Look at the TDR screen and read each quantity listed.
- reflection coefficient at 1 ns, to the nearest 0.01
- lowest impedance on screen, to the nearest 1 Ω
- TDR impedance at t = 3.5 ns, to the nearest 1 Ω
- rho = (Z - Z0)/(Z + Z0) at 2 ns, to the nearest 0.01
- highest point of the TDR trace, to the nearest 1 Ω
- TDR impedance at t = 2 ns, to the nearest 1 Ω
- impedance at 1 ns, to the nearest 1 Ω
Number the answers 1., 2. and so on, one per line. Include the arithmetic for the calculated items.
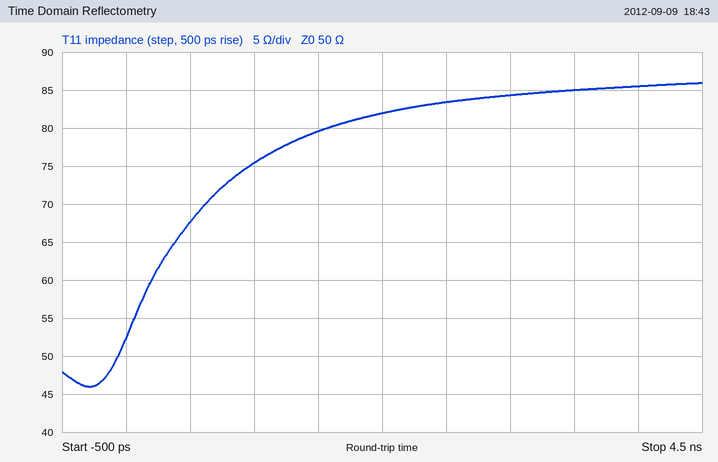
1. (75 − 50)/(75 + 50) ≈ +0.20
2. 46 Ω
3. 85 Ω
4. (82 − 50)/(82 + 50) ≈ +0.24
5. 86 Ω
6. 82 Ω
7. 75 Ω
